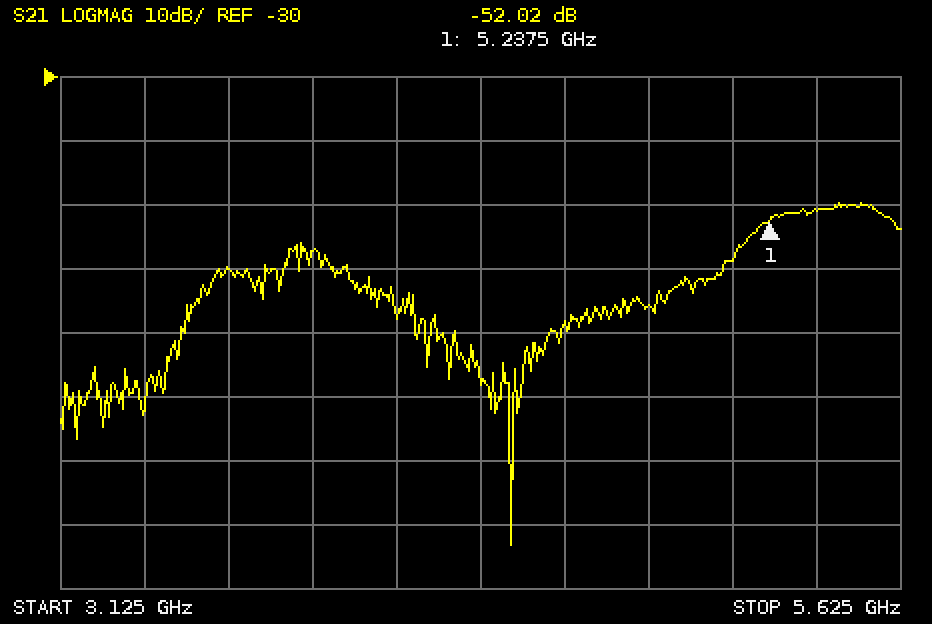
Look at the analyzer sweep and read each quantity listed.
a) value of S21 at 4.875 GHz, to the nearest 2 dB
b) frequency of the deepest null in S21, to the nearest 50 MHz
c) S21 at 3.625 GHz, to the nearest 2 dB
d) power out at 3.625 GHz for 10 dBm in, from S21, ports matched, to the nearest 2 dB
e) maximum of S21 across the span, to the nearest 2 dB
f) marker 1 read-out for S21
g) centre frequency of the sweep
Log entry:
-66 dB
4.45 GHz
-60 dB
-50 dBm
-50 dB
-52.02 dB
4.375 GHz
